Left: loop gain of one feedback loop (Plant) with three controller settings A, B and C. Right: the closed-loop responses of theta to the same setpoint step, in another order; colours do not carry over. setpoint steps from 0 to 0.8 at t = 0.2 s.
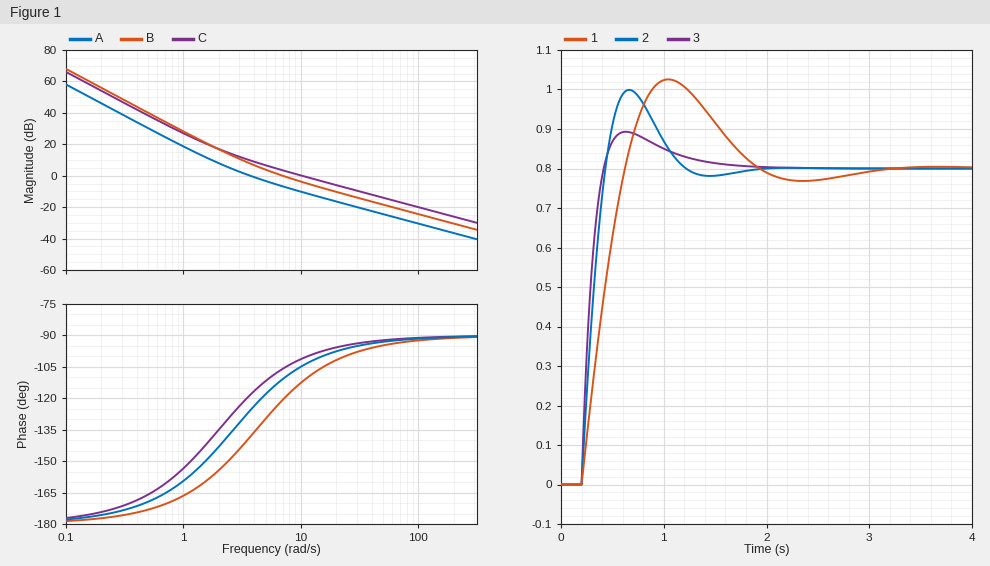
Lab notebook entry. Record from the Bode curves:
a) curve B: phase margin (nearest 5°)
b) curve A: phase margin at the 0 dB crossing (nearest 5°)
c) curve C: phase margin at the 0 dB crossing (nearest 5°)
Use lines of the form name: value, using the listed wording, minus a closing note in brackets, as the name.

curve B: phase margin: 60°
curve A: phase margin at the 0 dB crossing: 55°
curve C: phase margin at the 0 dB crossing: 80°
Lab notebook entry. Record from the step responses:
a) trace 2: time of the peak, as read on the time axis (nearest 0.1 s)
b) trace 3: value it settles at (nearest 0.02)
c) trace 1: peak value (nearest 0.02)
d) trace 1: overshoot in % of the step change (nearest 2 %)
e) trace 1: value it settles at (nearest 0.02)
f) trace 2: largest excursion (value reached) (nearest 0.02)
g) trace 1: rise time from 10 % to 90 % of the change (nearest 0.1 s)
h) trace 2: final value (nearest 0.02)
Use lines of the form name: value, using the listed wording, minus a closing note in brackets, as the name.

trace 2: time of the peak, as read on the time axis: 0.7 s
trace 3: value it settles at: 0.80
trace 1: peak value: 1.02
trace 1: overshoot in % of the step change: 28 %
trace 1: value it settles at: 0.80
trace 2: largest excursion (value reached): 1.00
trace 1: rise time from 10 % to 90 % of the change: 0.3 s
trace 2: final value: 0.80
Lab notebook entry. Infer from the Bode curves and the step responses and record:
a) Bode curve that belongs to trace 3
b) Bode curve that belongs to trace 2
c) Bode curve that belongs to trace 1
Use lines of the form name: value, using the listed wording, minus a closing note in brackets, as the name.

Bode curve that belongs to trace 3: C
Bode curve that belongs to trace 2: B
Bode curve that belongs to trace 1: A
